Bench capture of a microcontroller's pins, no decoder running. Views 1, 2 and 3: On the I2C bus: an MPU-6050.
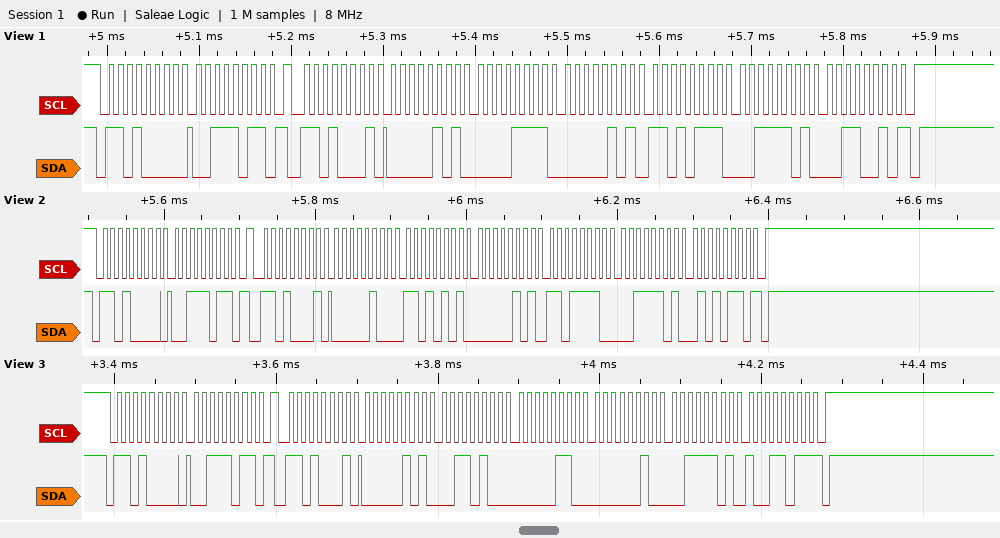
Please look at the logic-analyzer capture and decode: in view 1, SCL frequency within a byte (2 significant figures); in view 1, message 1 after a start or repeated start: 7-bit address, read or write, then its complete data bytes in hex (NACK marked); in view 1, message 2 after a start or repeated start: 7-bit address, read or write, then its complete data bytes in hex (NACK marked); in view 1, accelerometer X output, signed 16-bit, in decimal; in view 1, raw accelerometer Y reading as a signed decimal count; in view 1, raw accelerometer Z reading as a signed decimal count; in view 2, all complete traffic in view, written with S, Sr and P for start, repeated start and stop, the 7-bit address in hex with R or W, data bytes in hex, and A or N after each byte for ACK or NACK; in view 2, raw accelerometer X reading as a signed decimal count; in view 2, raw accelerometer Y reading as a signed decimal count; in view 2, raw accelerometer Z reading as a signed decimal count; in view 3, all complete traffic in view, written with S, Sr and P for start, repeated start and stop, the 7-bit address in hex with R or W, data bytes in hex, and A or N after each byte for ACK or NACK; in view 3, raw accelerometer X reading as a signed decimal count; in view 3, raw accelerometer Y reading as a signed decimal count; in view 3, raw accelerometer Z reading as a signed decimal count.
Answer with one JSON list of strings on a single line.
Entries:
["100 kHz", "0x68 write: 3B", "0x68 read: 05 0F 05 D7 3D 32 NACK", "1295", "1495", "15666", "S 68W A 3B A Sr 68R A 04 A D5 A 05 A DE A 3D A 56 N P", "1237", "1502", "15702", "S 68W A 3B A Sr 68R A 05 A 34 A 06 A 02 A 3D A 9B N P", "1332", "1538", "15771"]
